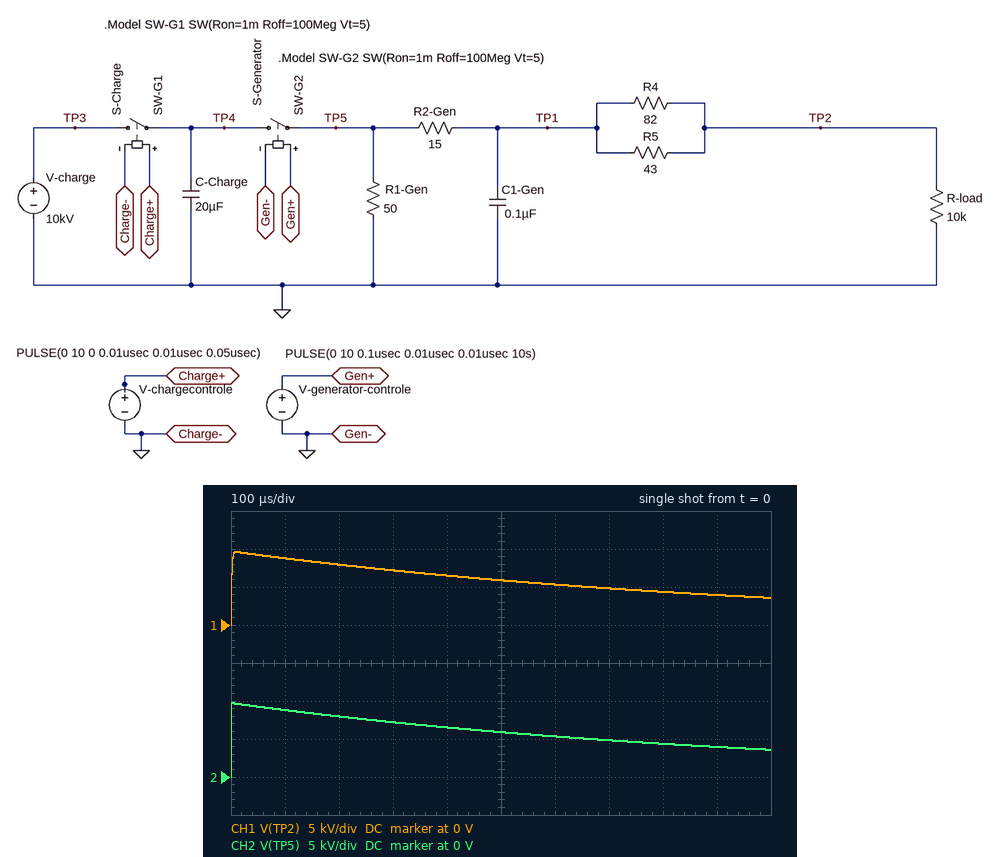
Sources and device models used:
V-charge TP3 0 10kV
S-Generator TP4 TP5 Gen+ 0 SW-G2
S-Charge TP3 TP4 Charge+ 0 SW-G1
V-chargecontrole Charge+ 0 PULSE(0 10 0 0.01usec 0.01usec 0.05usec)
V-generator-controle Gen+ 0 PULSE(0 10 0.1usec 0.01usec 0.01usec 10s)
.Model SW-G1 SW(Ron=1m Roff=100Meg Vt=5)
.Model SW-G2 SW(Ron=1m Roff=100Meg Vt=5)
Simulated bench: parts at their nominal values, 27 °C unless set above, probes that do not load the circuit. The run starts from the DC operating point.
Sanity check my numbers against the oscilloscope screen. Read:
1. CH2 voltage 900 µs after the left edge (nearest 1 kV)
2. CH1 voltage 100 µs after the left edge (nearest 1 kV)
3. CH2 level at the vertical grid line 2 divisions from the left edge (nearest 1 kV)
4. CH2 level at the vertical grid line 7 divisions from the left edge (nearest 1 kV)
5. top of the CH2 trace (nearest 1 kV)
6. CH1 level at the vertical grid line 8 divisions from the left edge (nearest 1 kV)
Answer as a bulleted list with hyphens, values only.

- 4 kV
- 9 kV
- 8 kV
- 5 kV
- 10 kV
- 4 kV
